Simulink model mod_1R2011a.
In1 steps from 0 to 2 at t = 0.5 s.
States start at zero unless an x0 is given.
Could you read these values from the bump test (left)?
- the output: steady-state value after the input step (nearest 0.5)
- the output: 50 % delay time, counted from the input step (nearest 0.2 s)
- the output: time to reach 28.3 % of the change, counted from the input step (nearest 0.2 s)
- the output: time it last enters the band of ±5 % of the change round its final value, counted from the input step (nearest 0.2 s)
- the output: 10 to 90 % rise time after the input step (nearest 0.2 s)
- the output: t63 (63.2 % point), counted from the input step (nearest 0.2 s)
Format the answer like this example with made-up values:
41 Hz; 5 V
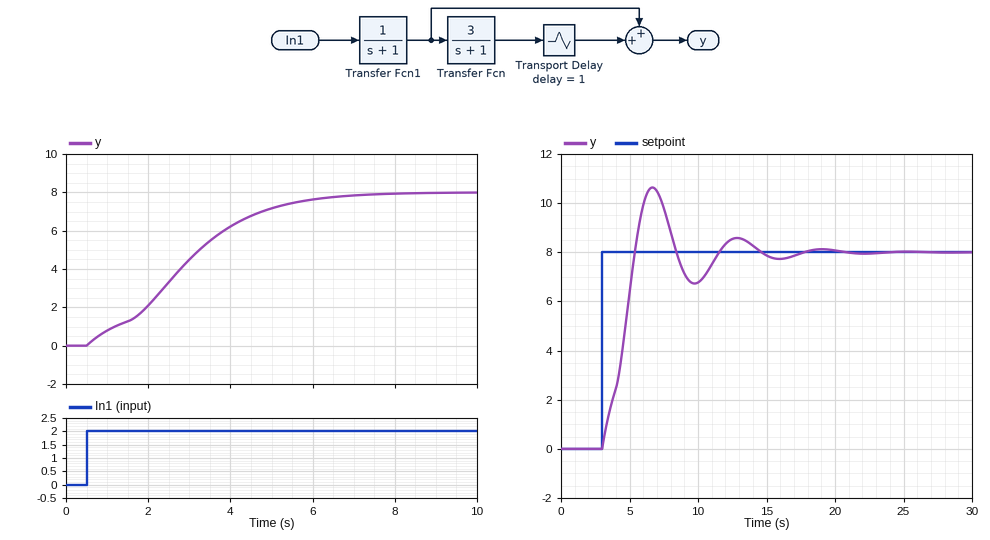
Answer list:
8.0; 2.2 s; 1.6 s; 5.4 s; 4.0 s; 2.8 s
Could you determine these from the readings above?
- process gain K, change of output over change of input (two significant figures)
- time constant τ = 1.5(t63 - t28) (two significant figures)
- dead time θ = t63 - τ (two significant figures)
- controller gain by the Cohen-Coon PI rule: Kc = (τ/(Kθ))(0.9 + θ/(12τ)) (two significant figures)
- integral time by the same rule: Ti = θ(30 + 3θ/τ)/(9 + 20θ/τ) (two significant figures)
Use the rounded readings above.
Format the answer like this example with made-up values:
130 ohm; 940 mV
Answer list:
4.0; 1.8 s; 1.0 s; 0.43; 1.6 s
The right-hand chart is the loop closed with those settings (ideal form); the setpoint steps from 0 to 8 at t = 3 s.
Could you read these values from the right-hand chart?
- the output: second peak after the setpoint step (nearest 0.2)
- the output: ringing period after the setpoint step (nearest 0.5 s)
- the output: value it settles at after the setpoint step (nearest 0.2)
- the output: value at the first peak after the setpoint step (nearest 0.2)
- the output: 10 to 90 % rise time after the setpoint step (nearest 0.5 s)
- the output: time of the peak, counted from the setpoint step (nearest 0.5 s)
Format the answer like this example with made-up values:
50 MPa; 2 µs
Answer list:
8.6; 6.0 s; 8.0; 10.6; 2.0 s; 3.5 s
